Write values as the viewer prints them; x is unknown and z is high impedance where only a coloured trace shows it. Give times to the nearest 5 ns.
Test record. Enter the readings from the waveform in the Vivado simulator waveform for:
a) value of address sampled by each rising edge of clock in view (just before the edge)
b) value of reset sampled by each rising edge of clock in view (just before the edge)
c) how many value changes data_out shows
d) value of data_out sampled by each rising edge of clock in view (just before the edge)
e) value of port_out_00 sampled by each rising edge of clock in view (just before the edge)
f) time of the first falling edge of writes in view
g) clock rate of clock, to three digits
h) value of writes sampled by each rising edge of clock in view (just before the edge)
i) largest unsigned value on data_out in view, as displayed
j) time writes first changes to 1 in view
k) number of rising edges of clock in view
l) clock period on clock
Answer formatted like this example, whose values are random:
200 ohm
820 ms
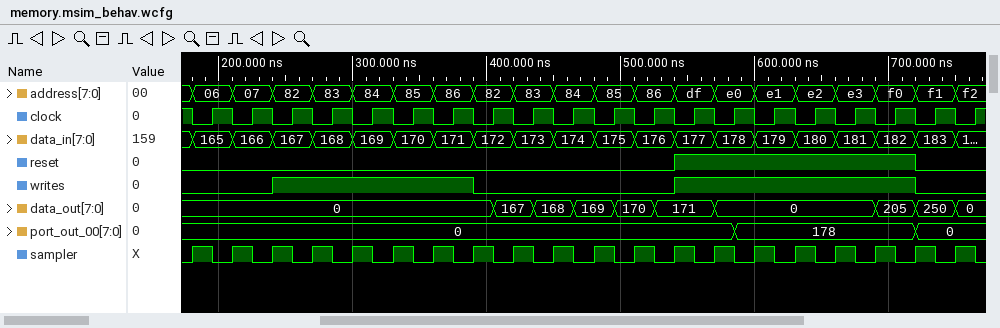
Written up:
06, 07, 82, 83, 84, 85, 86, 82, 83, 84, 85, 86, df, e0, e1, e2, e3, f0, f1, f2
0 0 0 0 0 0 0 0 0 0 0 0 1 1 1 1 1 1 0 0
9
0, 0, 0, 0, 0, 0, 0, 0, 167, 168, 169, 170, 171, 0, 0, 0, 0, 205, 250, 0
0, 0, 0, 0, 0, 0, 0, 0, 0, 0, 0, 0, 0, 0, 178, 178, 178, 178, 0, 0
390 ns
33.3 MHz
0 0 1 1 1 1 1 0 0 0 0 0 1 1 1 1 1 1 0 0
250
240 ns
20
30 ns
